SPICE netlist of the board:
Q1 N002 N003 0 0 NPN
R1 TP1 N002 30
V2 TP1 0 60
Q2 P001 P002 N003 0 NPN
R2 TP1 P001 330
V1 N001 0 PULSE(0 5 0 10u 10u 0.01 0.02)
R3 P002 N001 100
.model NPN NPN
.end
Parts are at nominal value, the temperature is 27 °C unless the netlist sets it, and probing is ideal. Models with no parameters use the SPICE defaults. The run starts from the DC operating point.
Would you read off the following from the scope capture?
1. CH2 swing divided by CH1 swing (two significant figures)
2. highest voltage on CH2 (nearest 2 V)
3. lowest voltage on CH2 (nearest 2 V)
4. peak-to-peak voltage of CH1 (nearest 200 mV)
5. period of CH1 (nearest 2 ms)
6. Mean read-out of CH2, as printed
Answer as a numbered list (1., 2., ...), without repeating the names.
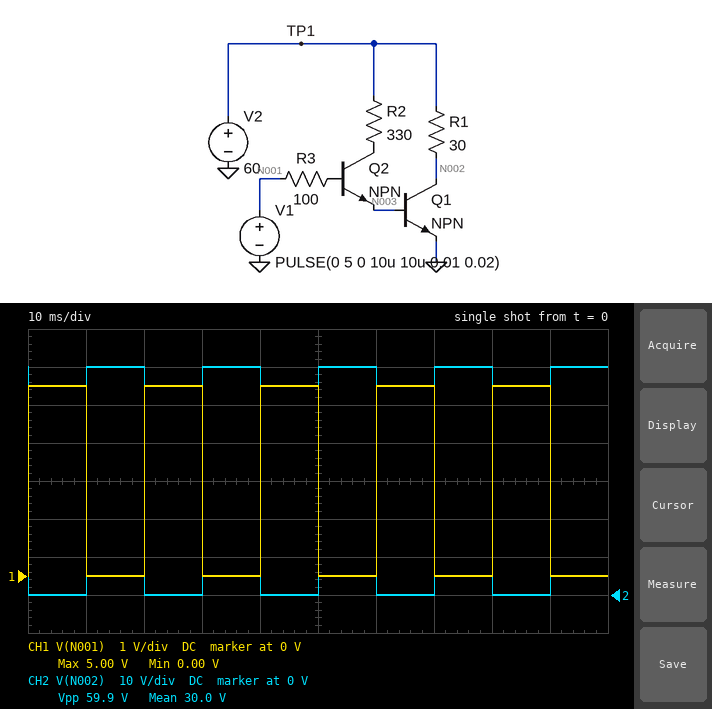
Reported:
1. 12
2. 60 V
3. 0 V
4. 5.0 V
5. 20 ms
6. 30.0 V
